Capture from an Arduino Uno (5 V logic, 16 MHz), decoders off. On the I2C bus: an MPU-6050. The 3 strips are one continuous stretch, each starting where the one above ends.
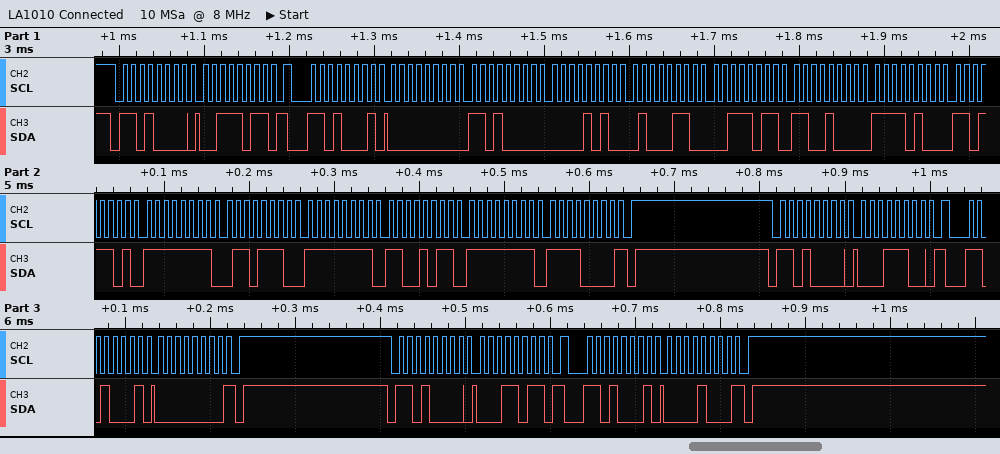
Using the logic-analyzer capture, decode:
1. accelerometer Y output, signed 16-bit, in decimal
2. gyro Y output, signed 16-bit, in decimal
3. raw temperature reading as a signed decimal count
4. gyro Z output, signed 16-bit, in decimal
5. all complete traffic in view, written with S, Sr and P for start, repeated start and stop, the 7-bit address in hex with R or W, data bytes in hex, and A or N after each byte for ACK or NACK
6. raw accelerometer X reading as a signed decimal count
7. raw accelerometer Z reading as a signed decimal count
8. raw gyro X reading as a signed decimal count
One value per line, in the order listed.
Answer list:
2630
-53
-2851
-16
S 68W A 3B A Sr 68R A 00 A D0 A 0A A 46 A 3B A C8 A F4 A DD A FF A 6E A FF A CB A FF A F0 N P S 68W A 1C A Sr 68R A 00 N P S 68W A 1B A Sr 68R A 08 N P
208
15304
-146
